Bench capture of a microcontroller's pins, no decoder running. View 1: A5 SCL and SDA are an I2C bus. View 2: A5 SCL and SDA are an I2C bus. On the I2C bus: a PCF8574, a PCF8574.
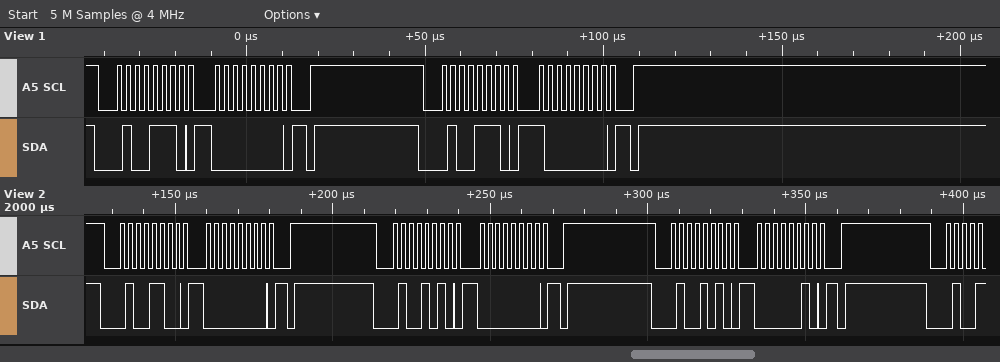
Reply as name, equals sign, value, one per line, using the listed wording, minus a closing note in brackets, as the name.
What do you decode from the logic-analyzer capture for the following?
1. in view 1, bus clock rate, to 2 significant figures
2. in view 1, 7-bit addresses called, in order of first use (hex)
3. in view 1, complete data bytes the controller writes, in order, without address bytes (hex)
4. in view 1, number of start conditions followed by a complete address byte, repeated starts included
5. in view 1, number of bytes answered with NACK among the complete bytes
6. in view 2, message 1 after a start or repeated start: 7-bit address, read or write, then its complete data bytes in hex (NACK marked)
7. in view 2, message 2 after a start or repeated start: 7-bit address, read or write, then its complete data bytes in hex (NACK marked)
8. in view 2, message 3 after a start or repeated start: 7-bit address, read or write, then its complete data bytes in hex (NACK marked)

in view 1, bus clock rate, to 2 significant figures = 400 kHz
in view 1, 7-bit addresses called, in order of first use = 0x27
in view 1, complete data bytes the controller writes, in order, without address bytes = 00 80
in view 1, number of start conditions followed by a complete address byte, repeated starts included = 2
in view 1, number of bytes answered with NACK among the complete bytes = 0
in view 2, message 1 after a start or repeated start: 7-bit address, read or write, then its complete data bytes in hex = 0x26 write: 00
in view 2, message 2 after a start or repeated start: 7-bit address, read or write, then its complete data bytes in hex = 0x25 write: 00
in view 2, message 3 after a start or repeated start: 7-bit address, read or write, then its complete data bytes in hex = 0x25 write: 02
